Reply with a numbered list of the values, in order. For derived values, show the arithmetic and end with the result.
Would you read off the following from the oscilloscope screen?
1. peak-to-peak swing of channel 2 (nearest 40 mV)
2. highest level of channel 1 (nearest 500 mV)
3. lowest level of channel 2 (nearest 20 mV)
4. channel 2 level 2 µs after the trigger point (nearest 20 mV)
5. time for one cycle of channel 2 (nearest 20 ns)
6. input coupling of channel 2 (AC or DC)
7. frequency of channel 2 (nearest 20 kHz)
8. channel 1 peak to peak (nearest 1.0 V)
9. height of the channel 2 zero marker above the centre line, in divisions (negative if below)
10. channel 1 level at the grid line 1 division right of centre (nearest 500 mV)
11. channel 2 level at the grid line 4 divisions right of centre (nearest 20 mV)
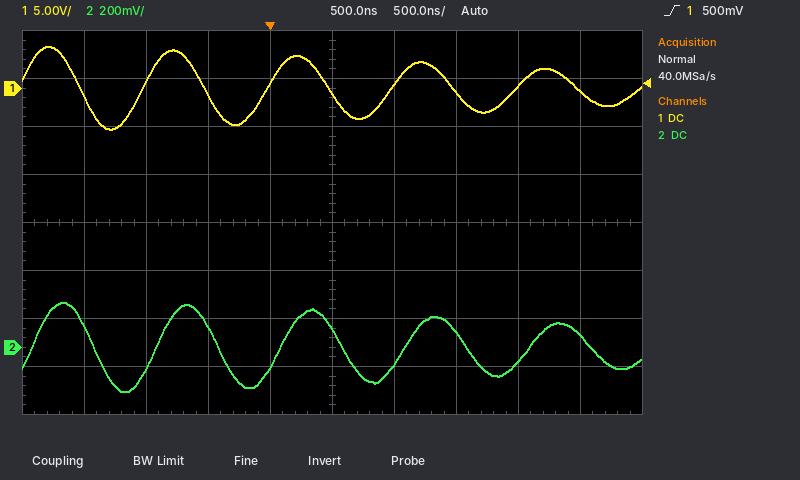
1. 360 mV
2. 4.5 V
3. -180 mV
4. -60 mV
5. 1.00 µs
6. DC
7. 1 / 1.00 µs ≈ 1.00 MHz
8. 9.0 V
9. -2.6 div
10. 500 mV
11. 60 mV
